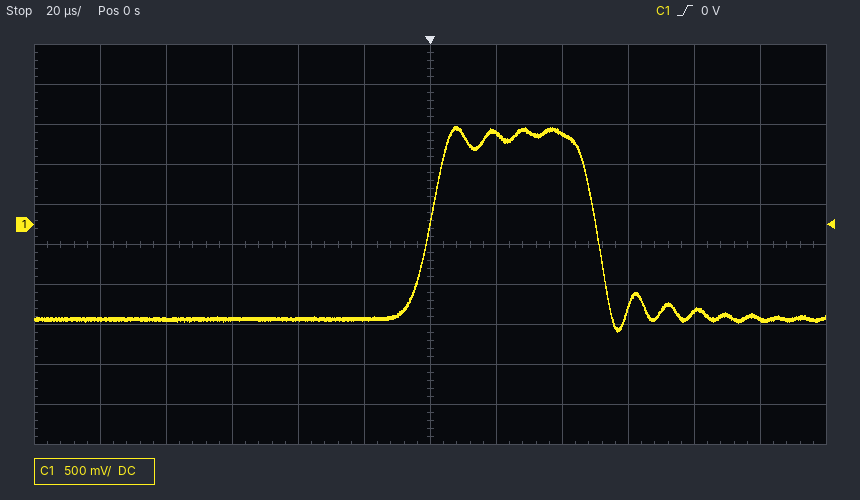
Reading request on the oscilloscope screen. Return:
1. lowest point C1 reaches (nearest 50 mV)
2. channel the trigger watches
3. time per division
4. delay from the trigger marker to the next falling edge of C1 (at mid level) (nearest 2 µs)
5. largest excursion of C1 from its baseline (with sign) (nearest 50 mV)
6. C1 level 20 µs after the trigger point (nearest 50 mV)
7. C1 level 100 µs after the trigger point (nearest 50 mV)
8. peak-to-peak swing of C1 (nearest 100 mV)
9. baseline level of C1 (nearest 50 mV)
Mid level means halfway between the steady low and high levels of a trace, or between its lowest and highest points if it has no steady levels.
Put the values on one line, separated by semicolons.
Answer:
-1.35 V; C1; 20 µs; 50 µs; +2.40 V; 1.15 V; -1.20 V; 2.60 V; -1.20 V
